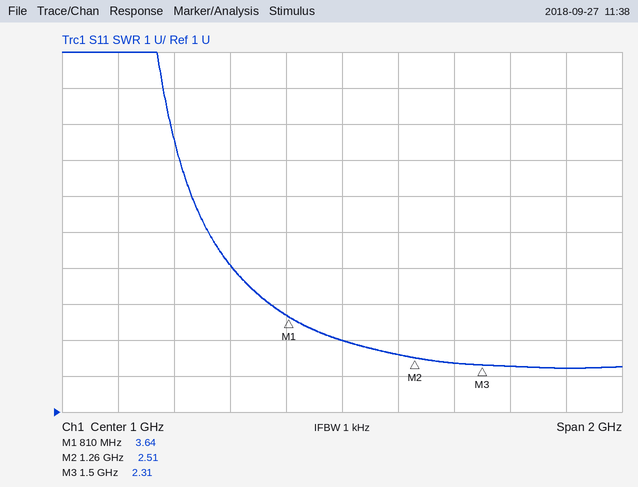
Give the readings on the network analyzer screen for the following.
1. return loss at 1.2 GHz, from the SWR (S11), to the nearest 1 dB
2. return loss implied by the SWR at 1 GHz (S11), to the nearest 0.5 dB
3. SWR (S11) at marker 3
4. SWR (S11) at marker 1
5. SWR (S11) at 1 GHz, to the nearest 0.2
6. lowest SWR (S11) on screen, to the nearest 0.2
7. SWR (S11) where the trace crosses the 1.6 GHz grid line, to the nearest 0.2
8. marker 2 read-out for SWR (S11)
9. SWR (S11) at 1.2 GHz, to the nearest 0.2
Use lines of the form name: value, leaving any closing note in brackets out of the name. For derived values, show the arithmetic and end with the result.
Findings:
return loss at 1.2 GHz, from the SWR (S11), to the nearest 1 dB: −20 log10((2.6 − 1)/(2.6 + 1)) ≈ 7 dB
return loss implied by the SWR at 1 GHz (S11), to the nearest 0.5 dB: −20 log10((3 − 1)/(3 + 1)) ≈ 6.0 dB
SWR (S11) at marker 3: 2.31
SWR (S11) at marker 1: 3.64
SWR (S11) at 1 GHz, to the nearest 0.2: 3.0
lowest SWR (S11) on screen, to the nearest 0.2: 2.2
SWR (S11) where the trace crosses the 1.6 GHz grid line, to the nearest 0.2: 2.2
marker 2 read-out for SWR: 2.51
SWR (S11) at 1.2 GHz, to the nearest 0.2: 2.6
